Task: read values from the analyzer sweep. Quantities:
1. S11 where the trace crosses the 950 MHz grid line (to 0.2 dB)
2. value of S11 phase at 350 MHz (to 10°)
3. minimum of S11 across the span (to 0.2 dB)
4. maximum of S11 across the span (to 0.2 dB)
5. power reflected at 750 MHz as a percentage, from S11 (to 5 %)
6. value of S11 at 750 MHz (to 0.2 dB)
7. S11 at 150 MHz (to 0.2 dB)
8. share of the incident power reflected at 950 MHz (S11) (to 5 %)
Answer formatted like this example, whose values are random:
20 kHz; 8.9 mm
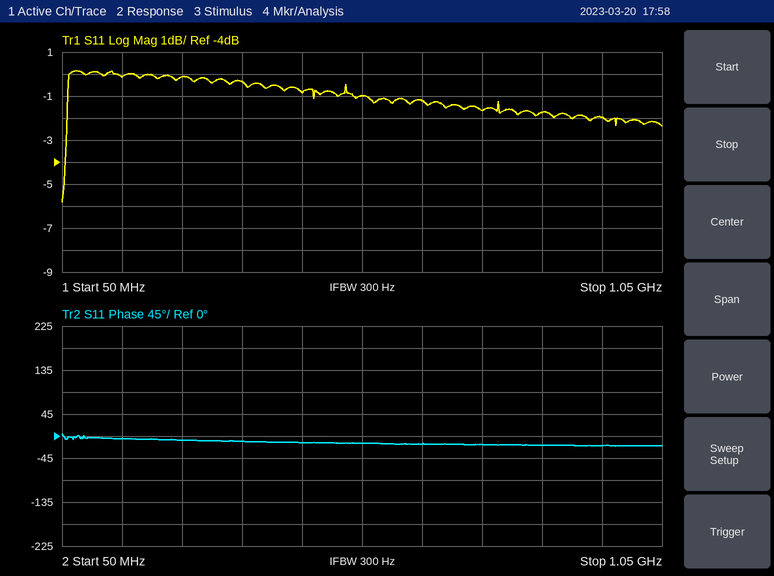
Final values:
-2.0 dB; -10°; -5.8 dB; 0.2 dB; 70 %; -1.6 dB; -0.2 dB; 65 %
